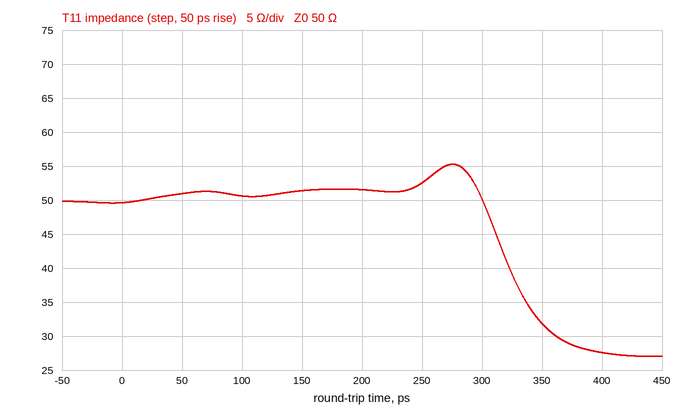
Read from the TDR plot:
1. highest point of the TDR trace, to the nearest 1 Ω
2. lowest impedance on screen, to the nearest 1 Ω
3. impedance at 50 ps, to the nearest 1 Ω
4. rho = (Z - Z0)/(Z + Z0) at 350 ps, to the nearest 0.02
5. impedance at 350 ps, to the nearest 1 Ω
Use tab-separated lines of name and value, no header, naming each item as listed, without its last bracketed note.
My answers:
highest point of the TDR trace, to the nearest 1 Ω	55 Ω
lowest impedance on screen, to the nearest 1 Ω	27 Ω
impedance at 50 ps, to the nearest 1 Ω	51 Ω
rho = (Z - Z0)/(Z + Z0) at 350 ps, to the nearest 0.02	-0.22
impedance at 350 ps, to the nearest 1 Ω	32 Ω
